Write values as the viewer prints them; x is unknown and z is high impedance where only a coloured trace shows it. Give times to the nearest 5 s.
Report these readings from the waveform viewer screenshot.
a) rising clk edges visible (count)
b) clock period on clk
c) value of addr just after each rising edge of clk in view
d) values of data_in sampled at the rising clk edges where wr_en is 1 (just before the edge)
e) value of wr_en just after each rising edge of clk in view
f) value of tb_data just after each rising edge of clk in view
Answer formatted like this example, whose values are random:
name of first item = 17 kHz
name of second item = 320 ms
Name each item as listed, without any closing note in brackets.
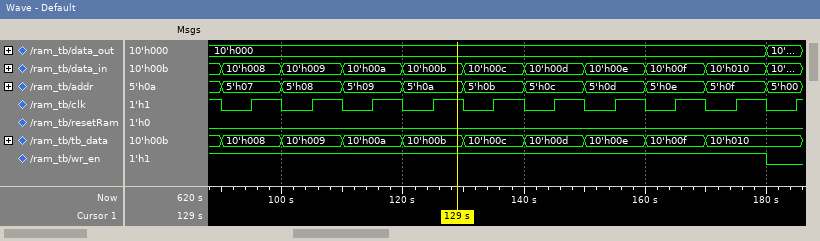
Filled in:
rising clk edges visible = 10
clock period on clk = 10 s
value of addr just after each rising edge of clk in view = 5'h07, 5'h08, 5'h09, 5'h0a, 5'h0b, 5'h0c, 5'h0d, 5'h0e, 5'h0f, 5'h00
values of data_in sampled at the rising clk edges where wr_en is 1 = 10'h008, 10'h009, 10'h00a, 10'h00b, 10'h00c, 10'h00d, 10'h00e, 10'h00f, 10'h010
value of wr_en just after each rising edge of clk in view = 1 1 1 1 1 1 1 1 1 0
value of tb_data just after each rising edge of clk in view = 10'h008, 10'h009, 10'h00a, 10'h00b, 10'h00c, 10'h00d, 10'h00e, 10'h00f, 10'h010, 10'h010
